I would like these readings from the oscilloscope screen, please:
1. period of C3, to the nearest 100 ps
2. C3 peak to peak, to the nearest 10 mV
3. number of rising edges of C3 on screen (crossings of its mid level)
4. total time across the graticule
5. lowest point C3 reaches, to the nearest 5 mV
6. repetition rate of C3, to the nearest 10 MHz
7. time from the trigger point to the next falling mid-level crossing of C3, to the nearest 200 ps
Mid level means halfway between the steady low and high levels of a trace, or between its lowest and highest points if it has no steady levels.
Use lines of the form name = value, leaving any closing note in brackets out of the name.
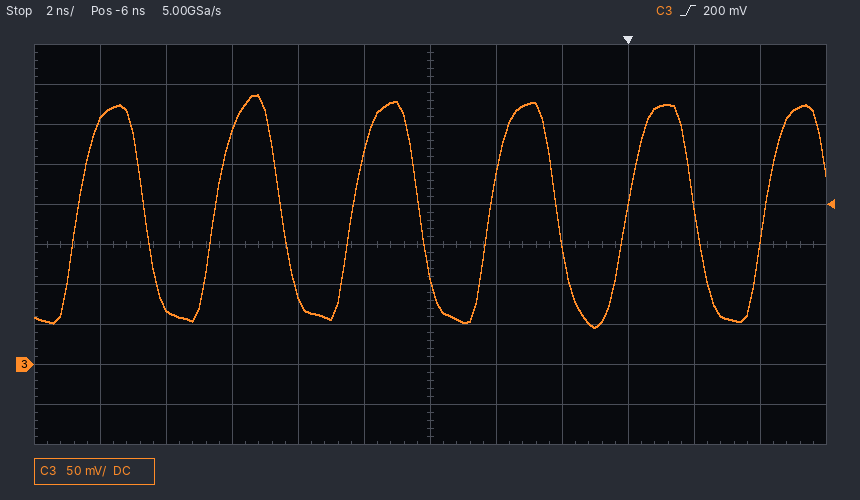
period of C3, to the nearest 100 ps = 4.2 ns
C3 peak to peak, to the nearest 10 mV = 290 mV
number of rising edges of C3 on screen = 6
total time across the graticule = 24 ns
lowest point C3 reaches, to the nearest 5 mV = 45 mV
repetition rate of C3, to the nearest 10 MHz = 240 MHz
time from the trigger point to the next falling mid-level crossing of C3, to the nearest 200 ps = 2.0 ns
